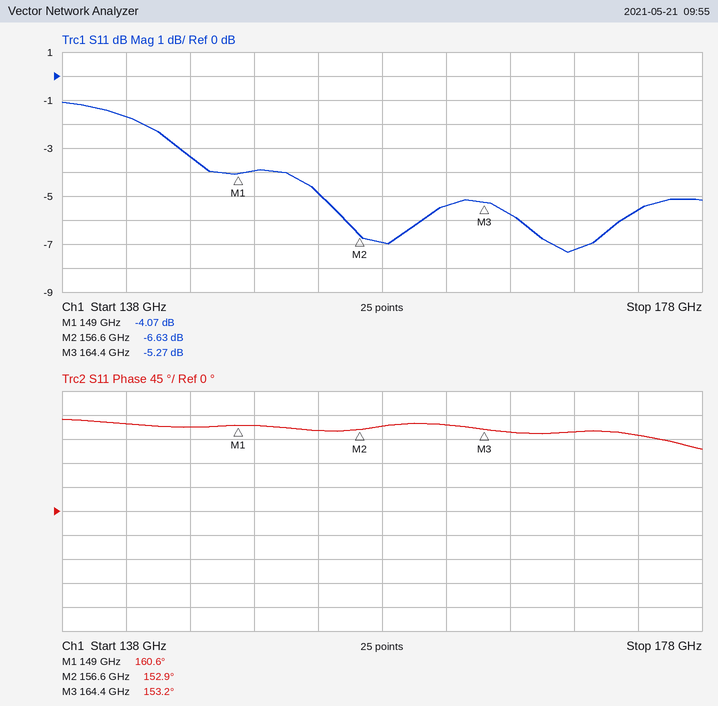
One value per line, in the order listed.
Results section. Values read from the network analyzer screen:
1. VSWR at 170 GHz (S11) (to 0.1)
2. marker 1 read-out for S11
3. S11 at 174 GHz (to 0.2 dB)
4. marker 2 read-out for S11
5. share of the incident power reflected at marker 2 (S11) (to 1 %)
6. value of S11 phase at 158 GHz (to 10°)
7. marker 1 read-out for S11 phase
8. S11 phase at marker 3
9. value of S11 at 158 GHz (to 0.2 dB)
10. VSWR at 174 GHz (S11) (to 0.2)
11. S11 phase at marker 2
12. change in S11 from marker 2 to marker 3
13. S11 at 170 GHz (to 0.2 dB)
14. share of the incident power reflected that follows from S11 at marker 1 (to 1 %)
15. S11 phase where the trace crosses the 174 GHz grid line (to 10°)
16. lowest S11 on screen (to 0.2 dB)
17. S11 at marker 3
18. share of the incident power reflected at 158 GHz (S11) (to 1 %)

2.5
-4.07 dB
-5.6 dB
-6.63 dB
22 %
160°
160.6°
153.2°
-7.0 dB
3.2
152.9°
1.36 dB
-7.2 dB
39 %
140°
-7.4 dB
-5.27 dB
20 %
